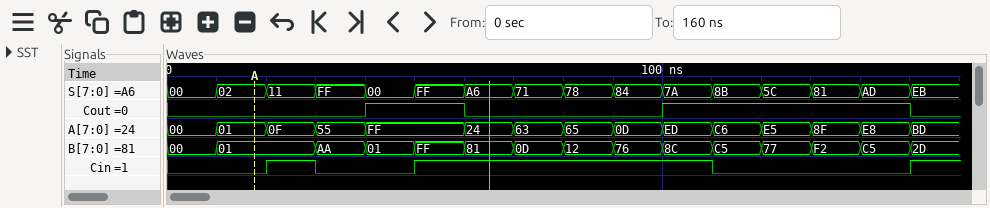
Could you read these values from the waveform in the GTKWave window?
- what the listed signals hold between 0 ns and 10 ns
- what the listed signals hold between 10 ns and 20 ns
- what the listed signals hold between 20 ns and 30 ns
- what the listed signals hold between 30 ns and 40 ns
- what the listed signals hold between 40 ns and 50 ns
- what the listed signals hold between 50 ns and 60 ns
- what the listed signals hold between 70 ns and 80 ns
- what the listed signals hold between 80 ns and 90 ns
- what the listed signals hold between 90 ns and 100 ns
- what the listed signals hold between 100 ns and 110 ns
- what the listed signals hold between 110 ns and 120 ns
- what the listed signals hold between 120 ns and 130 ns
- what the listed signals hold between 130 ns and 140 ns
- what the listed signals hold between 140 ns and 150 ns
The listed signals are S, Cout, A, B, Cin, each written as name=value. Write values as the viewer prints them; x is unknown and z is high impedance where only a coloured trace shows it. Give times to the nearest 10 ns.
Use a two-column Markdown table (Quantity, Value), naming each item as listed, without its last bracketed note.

| Quantity | Value |
|---|---|
| what the listed signals hold between 0 ns and 10 ns | S=00, Cout=0, A=00, B=00, Cin=0 |
| what the listed signals hold between 10 ns and 20 ns | S=02, Cout=0, A=01, B=01, Cin=0 |
| what the listed signals hold between 20 ns and 30 ns | S=11, Cout=0, A=0F, B=01, Cin=1 |
| what the listed signals hold between 30 ns and 40 ns | S=FF, Cout=0, A=55, B=AA, Cin=0 |
| what the listed signals hold between 40 ns and 50 ns | S=00, Cout=1, A=FF, B=01, Cin=0 |
| what the listed signals hold between 50 ns and 60 ns | S=FF, Cout=1, A=FF, B=FF, Cin=1 |
| what the listed signals hold between 70 ns and 80 ns | S=71, Cout=0, A=63, B=0D, Cin=1 |
| what the listed signals hold between 80 ns and 90 ns | S=78, Cout=0, A=65, B=12, Cin=1 |
| what the listed signals hold between 90 ns and 100 ns | S=84, Cout=0, A=0D, B=76, Cin=1 |
| what the listed signals hold between 100 ns and 110 ns | S=7A, Cout=1, A=ED, B=8C, Cin=1 |
| what the listed signals hold between 110 ns and 120 ns | S=8B, Cout=1, A=C6, B=C5, Cin=0 |
| what the listed signals hold between 120 ns and 130 ns | S=5C, Cout=1, A=E5, B=77, Cin=0 |
| what the listed signals hold between 130 ns and 140 ns | S=81, Cout=1, A=8F, B=F2, Cin=0 |
| what the listed signals hold between 140 ns and 150 ns | S=AD, Cout=1, A=E8, B=C5, Cin=0 |
